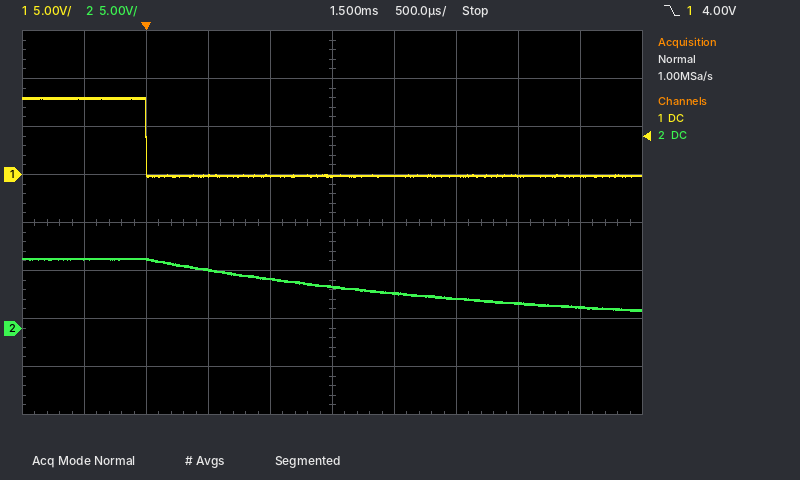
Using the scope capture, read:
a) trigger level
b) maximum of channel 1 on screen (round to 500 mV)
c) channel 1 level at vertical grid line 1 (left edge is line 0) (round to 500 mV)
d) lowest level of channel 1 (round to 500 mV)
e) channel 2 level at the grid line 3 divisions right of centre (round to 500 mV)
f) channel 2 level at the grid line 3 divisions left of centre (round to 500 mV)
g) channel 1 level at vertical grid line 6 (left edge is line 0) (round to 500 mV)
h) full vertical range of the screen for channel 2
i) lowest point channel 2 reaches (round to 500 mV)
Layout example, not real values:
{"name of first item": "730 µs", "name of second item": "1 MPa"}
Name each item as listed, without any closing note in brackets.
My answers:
{"trigger level": "4.00 V", "maximum of channel 1 on screen": "8.0 V", "channel 1 level at vertical grid line 1 (left edge is line 0)": "8.0 V", "lowest level of channel 1": "0.0 V", "channel 2 level at the grid line 3 divisions right of centre": "2.5 V", "channel 2 level at the grid line 3 divisions left of centre": "7.0 V", "channel 1 level at vertical grid line 6 (left edge is line 0)": "0.0 V", "full vertical range of the screen for channel 2": "40 V", "lowest point channel 2 reaches": "2.0 V"}
